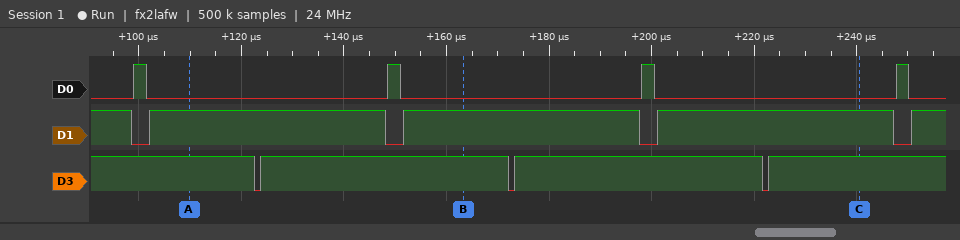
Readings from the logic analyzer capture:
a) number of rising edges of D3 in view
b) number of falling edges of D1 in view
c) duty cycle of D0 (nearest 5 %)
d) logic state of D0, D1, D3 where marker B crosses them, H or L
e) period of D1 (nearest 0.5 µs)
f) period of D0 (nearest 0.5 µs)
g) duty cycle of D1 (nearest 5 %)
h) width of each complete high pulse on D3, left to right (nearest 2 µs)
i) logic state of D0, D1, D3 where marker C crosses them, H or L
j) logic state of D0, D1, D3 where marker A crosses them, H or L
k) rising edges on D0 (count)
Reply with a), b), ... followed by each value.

a) 3
b) 4
c) 5 %
d) D0=L, D1=H, D3=H
e) 49.5 µs
f) 49.5 µs
g) 95 %
h) 48 µs, 48 µs
i) D0=L, D1=H, D3=H
j) D0=L, D1=H, D3=H
k) 4
